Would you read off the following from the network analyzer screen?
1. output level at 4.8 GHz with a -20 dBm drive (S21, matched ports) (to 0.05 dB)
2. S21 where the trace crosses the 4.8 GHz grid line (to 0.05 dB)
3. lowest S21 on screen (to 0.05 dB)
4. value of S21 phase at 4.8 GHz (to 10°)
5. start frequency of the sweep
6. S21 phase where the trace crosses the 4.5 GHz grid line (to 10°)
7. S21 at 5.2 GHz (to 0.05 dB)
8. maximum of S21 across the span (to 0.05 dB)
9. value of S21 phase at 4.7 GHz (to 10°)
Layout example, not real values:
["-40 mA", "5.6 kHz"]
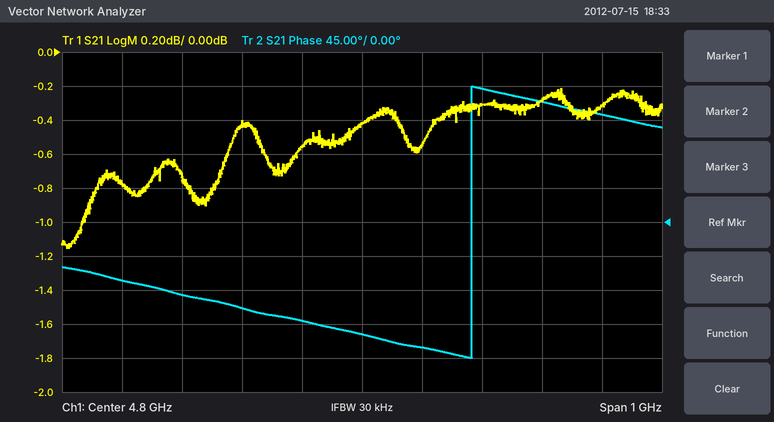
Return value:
["-20.40 dBm", "-0.40 dB", "-1.15 dB", "-150°", "4.3 GHz", "-100°", "-0.30 dB", "-0.20 dB", "-130°"]
